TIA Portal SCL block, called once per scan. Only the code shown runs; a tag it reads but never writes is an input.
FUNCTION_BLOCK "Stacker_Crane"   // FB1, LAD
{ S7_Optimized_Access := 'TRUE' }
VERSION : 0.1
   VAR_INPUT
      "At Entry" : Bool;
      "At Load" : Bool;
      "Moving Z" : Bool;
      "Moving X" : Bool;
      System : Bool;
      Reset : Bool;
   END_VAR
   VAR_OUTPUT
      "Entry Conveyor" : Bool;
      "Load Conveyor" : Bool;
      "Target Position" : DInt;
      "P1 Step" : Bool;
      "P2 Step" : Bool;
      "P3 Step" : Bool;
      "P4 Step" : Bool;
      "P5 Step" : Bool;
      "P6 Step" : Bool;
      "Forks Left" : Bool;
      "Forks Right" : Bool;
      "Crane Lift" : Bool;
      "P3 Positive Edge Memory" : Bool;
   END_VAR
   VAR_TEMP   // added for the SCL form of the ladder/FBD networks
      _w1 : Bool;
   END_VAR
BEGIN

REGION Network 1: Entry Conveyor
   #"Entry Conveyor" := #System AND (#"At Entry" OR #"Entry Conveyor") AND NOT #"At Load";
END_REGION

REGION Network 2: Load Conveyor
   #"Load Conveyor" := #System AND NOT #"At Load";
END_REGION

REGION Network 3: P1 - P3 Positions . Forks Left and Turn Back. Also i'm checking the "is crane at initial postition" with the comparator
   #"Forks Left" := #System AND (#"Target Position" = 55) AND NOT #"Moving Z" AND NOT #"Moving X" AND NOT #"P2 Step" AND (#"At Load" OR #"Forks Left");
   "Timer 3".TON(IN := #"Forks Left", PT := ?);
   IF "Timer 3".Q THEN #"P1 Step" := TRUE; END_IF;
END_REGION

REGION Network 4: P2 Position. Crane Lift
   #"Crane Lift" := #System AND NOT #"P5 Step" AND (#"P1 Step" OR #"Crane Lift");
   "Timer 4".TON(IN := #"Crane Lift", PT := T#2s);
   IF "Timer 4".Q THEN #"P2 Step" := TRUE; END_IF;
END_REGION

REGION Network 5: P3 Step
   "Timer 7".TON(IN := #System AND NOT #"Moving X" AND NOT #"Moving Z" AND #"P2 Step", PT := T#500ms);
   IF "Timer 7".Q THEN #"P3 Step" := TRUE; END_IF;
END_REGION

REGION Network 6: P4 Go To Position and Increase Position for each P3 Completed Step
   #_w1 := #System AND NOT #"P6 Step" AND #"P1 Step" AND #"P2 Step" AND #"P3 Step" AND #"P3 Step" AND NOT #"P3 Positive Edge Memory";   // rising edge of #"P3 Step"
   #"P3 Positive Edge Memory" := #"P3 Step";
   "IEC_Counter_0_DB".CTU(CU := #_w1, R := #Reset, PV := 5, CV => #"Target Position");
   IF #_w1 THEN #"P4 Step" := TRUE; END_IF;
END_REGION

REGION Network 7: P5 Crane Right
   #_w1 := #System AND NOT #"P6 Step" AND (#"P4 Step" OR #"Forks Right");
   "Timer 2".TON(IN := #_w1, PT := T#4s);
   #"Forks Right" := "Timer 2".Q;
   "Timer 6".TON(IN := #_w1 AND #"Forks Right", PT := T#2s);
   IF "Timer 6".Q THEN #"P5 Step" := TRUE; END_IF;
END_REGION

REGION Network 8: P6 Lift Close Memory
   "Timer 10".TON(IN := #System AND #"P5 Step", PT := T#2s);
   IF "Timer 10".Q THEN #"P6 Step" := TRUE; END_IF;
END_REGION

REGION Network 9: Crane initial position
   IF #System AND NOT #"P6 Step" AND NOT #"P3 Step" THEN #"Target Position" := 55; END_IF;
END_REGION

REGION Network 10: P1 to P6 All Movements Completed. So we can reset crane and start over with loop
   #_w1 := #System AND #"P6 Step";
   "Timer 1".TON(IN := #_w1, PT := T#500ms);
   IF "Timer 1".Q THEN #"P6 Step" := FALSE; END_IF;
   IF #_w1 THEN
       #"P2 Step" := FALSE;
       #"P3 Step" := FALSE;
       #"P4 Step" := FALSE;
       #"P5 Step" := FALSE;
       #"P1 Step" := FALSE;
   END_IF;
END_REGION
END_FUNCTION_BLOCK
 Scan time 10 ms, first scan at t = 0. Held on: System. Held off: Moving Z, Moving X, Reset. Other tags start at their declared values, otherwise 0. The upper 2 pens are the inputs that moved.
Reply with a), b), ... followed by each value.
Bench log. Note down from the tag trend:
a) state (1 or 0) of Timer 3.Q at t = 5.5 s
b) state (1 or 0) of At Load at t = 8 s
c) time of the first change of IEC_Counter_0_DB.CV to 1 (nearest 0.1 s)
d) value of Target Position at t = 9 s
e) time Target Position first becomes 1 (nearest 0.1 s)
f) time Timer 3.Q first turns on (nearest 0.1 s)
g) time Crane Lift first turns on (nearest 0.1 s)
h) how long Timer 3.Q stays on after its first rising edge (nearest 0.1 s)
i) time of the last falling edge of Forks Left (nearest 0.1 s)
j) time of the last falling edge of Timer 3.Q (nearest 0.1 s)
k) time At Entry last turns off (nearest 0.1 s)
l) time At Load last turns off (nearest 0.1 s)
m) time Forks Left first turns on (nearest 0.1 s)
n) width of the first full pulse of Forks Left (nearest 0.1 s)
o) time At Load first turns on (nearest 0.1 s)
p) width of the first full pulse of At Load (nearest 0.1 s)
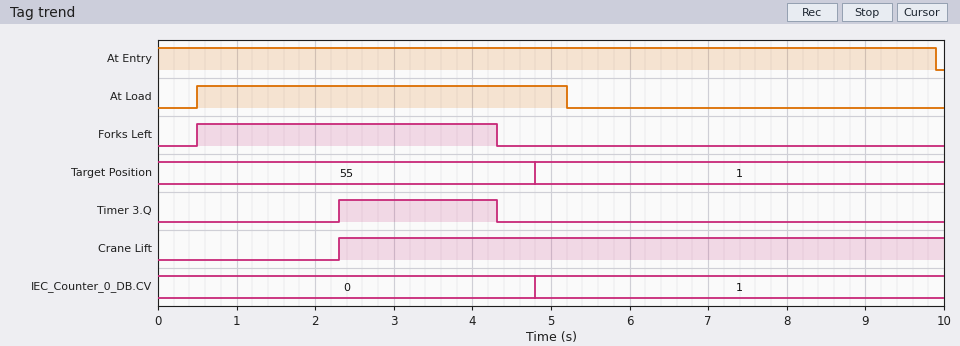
a) 0
b) 0
c) 4.8 s
d) 1
e) 4.8 s
f) 2.3 s
g) 2.3 s
h) 2.0 s
i) 4.3 s
j) 4.3 s
k) 9.9 s
l) 5.2 s
m) 0.5 s
n) 3.8 s
o) 0.5 s
p) 4.7 s
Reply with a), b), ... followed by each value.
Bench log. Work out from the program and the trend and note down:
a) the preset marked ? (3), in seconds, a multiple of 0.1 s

a) 1.8 s
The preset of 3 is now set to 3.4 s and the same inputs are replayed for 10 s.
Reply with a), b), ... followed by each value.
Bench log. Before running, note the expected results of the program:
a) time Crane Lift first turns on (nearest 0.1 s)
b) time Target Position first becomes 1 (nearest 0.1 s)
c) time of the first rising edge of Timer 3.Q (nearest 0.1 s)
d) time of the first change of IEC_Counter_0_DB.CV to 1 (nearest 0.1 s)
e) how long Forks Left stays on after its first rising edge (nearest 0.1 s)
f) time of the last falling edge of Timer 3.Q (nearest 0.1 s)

a) 3.9 s
b) 6.4 s
c) 3.9 s
d) 6.4 s
e) 5.4 s
f) 5.9 s
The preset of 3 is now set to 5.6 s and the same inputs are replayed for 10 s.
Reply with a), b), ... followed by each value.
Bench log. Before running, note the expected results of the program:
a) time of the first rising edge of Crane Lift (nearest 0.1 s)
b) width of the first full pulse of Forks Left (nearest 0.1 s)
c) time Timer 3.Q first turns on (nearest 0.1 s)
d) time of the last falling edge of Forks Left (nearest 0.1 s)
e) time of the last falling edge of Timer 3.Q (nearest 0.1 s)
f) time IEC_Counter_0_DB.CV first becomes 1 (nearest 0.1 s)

a) 6.1 s
b) 7.6 s
c) 6.1 s
d) 8.1 s
e) 8.1 s
f) 8.6 s
